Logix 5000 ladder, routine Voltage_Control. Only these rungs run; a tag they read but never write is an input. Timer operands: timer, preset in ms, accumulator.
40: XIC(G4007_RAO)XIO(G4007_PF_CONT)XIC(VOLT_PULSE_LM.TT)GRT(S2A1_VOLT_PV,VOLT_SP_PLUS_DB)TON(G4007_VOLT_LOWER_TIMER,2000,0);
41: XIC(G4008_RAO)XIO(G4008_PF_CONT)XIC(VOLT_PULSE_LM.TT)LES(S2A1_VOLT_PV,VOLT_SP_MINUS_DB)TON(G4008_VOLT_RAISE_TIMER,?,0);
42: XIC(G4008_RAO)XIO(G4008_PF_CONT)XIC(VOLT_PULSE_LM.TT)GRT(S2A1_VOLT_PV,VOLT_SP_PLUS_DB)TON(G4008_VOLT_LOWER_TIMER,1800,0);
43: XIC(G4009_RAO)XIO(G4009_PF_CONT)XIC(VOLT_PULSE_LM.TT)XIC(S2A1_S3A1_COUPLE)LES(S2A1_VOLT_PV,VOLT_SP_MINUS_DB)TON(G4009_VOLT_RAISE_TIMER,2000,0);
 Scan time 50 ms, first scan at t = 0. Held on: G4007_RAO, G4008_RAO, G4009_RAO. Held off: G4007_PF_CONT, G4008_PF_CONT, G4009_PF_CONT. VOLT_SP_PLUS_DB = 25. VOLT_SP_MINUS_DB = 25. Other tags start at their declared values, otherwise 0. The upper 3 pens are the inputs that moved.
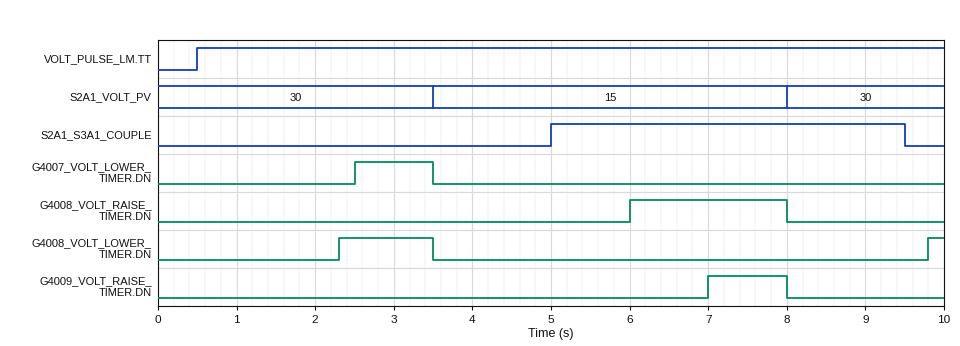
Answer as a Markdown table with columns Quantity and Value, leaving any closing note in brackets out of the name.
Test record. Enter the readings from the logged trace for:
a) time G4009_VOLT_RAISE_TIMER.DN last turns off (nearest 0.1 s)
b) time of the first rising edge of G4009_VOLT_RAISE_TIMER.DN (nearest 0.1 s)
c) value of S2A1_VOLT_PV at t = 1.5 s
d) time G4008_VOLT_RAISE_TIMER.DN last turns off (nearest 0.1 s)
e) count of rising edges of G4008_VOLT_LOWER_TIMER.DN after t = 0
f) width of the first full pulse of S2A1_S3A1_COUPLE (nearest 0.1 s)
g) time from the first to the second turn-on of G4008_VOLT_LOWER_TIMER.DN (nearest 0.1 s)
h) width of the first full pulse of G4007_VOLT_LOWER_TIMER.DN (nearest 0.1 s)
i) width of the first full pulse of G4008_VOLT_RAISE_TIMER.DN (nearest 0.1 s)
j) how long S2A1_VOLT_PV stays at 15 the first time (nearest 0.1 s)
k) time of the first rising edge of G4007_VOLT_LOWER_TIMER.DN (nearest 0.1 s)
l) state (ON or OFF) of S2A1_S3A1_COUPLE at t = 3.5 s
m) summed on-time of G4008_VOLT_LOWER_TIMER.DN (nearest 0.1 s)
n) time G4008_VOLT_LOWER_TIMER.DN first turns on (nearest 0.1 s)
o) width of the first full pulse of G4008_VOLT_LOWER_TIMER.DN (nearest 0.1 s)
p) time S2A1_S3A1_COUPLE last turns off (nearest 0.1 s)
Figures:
| Quantity | Value |
|---|---|
| time G4009_VOLT_RAISE_TIMER.DN last turns off | 8.0 s |
| time of the first rising edge of G4009_VOLT_RAISE_TIMER.DN | 7.0 s |
| value of S2A1_VOLT_PV at t = 1.5 s | 30 |
| time G4008_VOLT_RAISE_TIMER.DN last turns off | 8.0 s |
| count of rising edges of G4008_VOLT_LOWER_TIMER.DN after t = 0 | 2 |
| width of the first full pulse of S2A1_S3A1_COUPLE | 4.5 s |
| time from the first to the second turn-on of G4008_VOLT_LOWER_TIMER.DN | 7.5 s |
| width of the first full pulse of G4007_VOLT_LOWER_TIMER.DN | 1.0 s |
| width of the first full pulse of G4008_VOLT_RAISE_TIMER.DN | 2.0 s |
| how long S2A1_VOLT_PV stays at 15 the first time | 4.5 s |
| time of the first rising edge of G4007_VOLT_LOWER_TIMER.DN | 2.5 s |
| state (ON or OFF) of S2A1_S3A1_COUPLE at t = 3.5 s | OFF |
| summed on-time of G4008_VOLT_LOWER_TIMER.DN | 1.4 s |
| time G4008_VOLT_LOWER_TIMER.DN first turns on | 2.3 s |
| width of the first full pulse of G4008_VOLT_LOWER_TIMER.DN | 1.2 s |
| time S2A1_S3A1_COUPLE last turns off | 9.5 s |
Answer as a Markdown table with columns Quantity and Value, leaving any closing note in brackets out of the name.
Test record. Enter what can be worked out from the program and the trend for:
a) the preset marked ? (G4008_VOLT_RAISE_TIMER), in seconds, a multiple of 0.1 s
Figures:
| Quantity | Value |
|---|---|
| the preset marked ? (G4008_VOLT_RAISE_TIMER), in seconds, a multiple of 0.1 s | 2.5 s |
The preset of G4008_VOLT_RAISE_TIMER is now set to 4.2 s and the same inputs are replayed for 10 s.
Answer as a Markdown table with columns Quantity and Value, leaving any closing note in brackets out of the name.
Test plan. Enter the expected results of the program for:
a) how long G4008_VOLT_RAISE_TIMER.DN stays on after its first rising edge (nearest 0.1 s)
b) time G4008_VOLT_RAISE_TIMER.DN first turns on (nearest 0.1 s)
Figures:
| Quantity | Value |
|---|---|
| how long G4008_VOLT_RAISE_TIMER.DN stays on after its first rising edge | 0.3 s |
| time G4008_VOLT_RAISE_TIMER.DN first turns on | 7.7 s |
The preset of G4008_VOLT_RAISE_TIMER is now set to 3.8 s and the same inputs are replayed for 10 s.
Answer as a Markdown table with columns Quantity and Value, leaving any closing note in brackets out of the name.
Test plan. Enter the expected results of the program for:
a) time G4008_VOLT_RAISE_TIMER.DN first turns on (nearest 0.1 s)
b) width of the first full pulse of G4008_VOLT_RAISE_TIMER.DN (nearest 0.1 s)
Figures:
| Quantity | Value |
|---|---|
| time G4008_VOLT_RAISE_TIMER.DN first turns on | 7.3 s |
| width of the first full pulse of G4008_VOLT_RAISE_TIMER.DN | 0.7 s |
